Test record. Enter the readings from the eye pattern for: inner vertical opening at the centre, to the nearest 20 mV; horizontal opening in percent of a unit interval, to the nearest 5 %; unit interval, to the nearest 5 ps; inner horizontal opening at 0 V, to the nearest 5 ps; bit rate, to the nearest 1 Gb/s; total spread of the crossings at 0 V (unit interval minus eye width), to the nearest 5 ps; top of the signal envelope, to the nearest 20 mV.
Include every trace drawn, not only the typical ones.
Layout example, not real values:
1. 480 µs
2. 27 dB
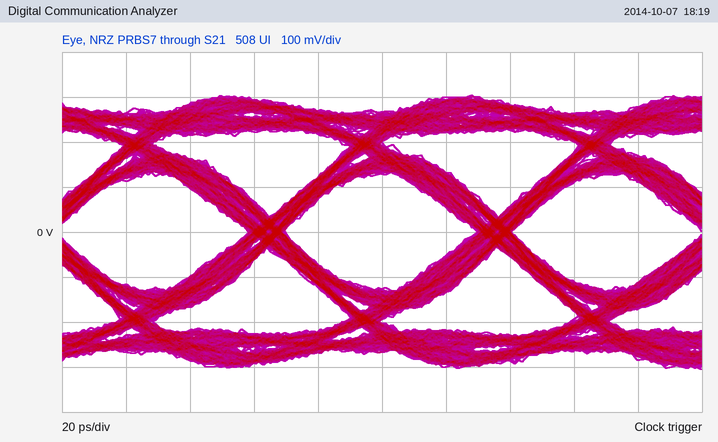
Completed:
1. 260 mV
2. 85 %
3. 70 ps
4. 60 ps
5. 14 Gb/s
6. 10 ps
7. 300 mV
